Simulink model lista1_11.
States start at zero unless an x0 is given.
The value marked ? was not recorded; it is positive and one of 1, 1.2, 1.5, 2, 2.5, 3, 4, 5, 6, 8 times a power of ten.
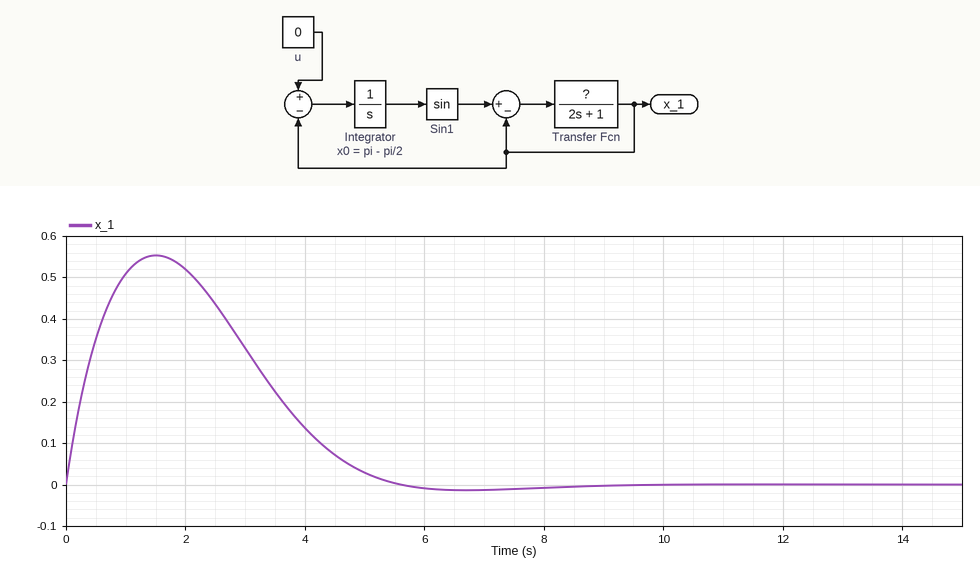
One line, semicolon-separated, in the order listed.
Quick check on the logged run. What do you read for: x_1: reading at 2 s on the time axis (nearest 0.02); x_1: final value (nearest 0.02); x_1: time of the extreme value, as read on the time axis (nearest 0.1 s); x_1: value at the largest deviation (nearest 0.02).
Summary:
0.52; 0.00; 1.5 s; 0.56
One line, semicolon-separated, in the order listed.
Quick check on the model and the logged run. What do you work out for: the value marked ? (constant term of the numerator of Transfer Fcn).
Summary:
2
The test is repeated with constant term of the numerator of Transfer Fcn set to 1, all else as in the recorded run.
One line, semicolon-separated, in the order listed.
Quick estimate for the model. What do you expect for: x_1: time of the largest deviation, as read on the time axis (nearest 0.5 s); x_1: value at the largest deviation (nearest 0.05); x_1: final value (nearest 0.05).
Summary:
2.0 s; 0.40; 0.00
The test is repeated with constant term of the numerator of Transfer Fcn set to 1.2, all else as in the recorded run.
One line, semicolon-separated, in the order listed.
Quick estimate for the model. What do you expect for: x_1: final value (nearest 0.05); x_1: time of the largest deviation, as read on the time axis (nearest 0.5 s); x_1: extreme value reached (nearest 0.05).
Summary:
0.00; 2.0 s; 0.45
